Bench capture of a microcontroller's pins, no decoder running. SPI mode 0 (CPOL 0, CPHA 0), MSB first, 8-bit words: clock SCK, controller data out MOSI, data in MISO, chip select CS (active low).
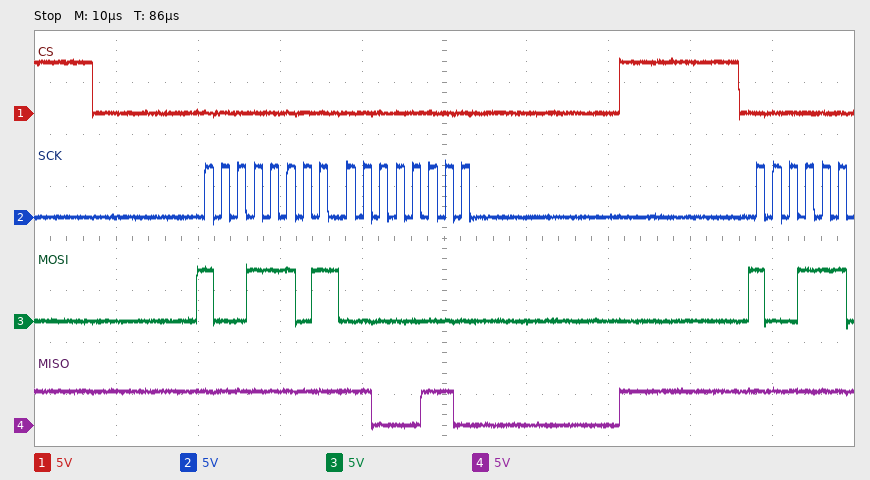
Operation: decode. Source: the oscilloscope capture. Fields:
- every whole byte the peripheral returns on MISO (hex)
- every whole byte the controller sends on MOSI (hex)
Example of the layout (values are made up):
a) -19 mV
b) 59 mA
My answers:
a) FF C6
b) 9D 00
